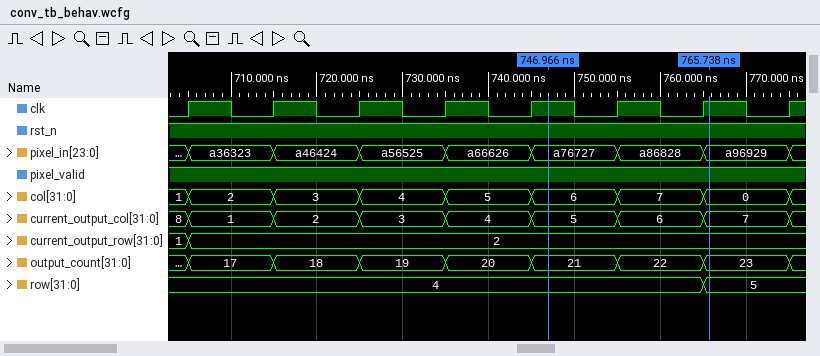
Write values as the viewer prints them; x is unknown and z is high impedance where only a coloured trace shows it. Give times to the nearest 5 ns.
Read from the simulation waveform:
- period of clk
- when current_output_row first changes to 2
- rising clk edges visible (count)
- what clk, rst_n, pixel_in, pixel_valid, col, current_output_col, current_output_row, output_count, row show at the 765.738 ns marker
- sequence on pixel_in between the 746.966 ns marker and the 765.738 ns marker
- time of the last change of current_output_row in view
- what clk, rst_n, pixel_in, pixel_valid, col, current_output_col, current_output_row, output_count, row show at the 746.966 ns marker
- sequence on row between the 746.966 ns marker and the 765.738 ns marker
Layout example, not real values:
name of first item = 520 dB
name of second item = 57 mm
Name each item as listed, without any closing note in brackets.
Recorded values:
period of clk = 10 ns
when current_output_row first changes to 2 = 705 ns
rising clk edges visible = 8
what clk, rst_n, pixel_in, pixel_valid, col, current_output_col, current_output_row, output_count, row show at the 765.738 ns marker = clk=1, rst_n=1, pixel_in=a96929, pixel_valid=1, col=0, current_output_col=7, current_output_row=2, output_count=23, row=5
sequence on pixel_in between the 746.966 ns marker and the 765.738 ns marker = a76727, a86828, a96929
time of the last change of current_output_row in view = 705 ns
what clk, rst_n, pixel_in, pixel_valid, col, current_output_col, current_output_row, output_count, row show at the 746.966 ns marker = clk=1, rst_n=1, pixel_in=a76727, pixel_valid=1, col=6, current_output_col=5, current_output_row=2, output_count=21, row=4
sequence on row between the 746.966 ns marker and the 765.738 ns marker = 4, 5
